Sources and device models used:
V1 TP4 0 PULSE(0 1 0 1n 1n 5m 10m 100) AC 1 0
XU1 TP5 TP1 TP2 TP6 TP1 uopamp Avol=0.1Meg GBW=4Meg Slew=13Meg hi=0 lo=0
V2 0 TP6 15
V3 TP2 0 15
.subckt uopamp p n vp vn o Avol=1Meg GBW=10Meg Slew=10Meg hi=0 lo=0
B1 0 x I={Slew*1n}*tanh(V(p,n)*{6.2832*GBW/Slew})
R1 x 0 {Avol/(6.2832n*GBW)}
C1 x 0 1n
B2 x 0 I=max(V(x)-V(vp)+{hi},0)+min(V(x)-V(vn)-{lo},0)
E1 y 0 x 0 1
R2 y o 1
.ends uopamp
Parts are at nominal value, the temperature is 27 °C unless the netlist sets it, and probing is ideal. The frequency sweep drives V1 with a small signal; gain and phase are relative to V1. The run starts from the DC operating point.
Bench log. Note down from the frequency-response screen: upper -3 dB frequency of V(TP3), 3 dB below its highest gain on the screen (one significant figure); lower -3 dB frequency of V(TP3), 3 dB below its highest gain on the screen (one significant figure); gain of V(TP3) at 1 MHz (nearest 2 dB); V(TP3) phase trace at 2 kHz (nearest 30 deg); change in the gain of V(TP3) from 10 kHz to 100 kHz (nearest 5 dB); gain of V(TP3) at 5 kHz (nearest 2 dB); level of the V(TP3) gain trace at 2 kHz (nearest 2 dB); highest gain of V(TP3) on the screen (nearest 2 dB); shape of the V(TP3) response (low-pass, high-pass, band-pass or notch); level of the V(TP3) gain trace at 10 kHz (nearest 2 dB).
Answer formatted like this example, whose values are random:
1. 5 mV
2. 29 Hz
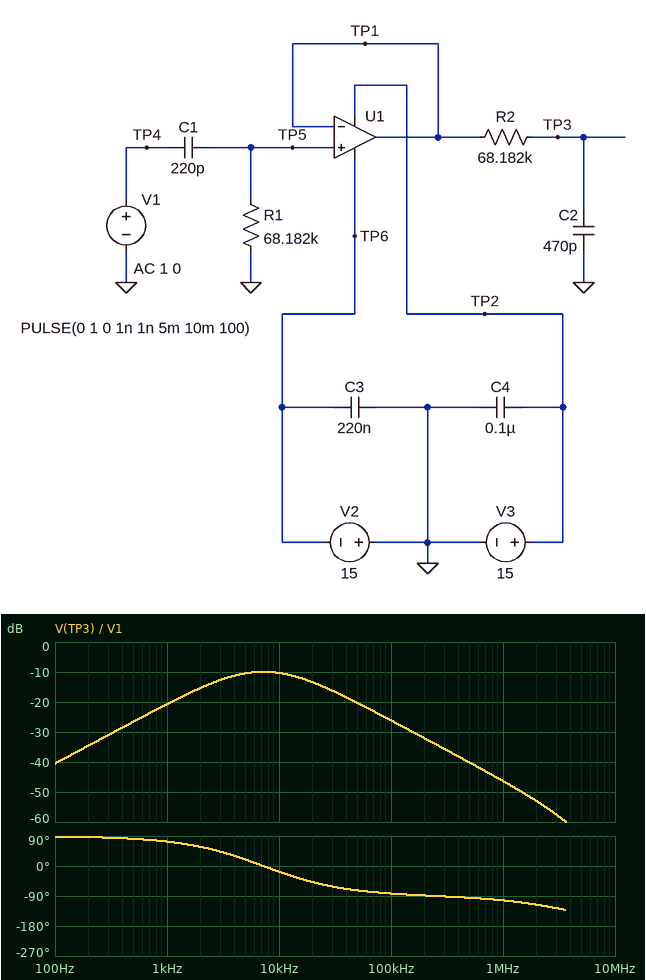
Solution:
1. 20 kHz
2. 3 kHz
3. -46 dB
4. 60 deg
5. -15 dB
6. -10 dB
7. -16 dB
8. -10 dB
9. band-pass
10. -10 dB
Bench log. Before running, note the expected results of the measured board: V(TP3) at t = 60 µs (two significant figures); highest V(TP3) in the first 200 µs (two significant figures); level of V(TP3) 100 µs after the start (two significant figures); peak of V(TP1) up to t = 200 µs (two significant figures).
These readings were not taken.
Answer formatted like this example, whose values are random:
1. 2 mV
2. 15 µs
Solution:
1. 120 mV
2. 240 mV
3. 38 mV
4. 990 mV
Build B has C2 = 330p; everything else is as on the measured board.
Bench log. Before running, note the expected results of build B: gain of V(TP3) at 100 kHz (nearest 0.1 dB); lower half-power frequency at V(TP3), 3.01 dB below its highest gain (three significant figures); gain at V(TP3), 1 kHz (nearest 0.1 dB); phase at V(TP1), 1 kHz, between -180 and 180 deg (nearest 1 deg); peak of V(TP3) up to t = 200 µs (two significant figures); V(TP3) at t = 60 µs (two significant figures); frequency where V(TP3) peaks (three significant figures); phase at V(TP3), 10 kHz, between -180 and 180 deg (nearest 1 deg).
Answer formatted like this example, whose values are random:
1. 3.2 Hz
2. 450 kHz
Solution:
1. -23.1 dB
2. 3.54 kHz
3. -20.6 dB
4. 85 deg
5. 300 mV
6. 100 mV
7. 8.66 kHz
8. -8 deg
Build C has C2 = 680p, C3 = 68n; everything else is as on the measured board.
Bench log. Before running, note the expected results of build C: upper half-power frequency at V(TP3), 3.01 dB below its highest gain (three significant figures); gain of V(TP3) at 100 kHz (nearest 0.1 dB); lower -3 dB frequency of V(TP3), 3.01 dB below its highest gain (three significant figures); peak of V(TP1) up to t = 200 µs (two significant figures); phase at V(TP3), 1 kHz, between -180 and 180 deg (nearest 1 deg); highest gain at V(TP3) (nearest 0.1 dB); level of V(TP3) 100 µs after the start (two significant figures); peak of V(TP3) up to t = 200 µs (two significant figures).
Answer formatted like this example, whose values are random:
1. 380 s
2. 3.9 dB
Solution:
1. 16.3 kHz
2. -29.3 dB
3. 2.24 kHz
4. 990 mV
5. 68 deg
6. -12.2 dB
7. 55 mV
8. 190 mV
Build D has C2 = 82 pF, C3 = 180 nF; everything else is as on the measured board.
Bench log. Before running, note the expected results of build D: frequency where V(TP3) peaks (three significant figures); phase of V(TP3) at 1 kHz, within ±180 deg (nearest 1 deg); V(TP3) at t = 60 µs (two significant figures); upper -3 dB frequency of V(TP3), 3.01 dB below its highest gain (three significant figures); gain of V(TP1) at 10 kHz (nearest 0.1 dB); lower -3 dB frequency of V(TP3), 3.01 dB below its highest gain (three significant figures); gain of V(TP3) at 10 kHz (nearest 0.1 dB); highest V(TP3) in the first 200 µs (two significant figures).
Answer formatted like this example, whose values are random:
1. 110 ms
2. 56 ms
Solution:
1. 17.4 kHz
2. 83 deg
3. 29 mV
4. 45.7 kHz
5. -3.3 dB
6. 6.61 kHz
7. -3.8 dB
8. 560 mV
